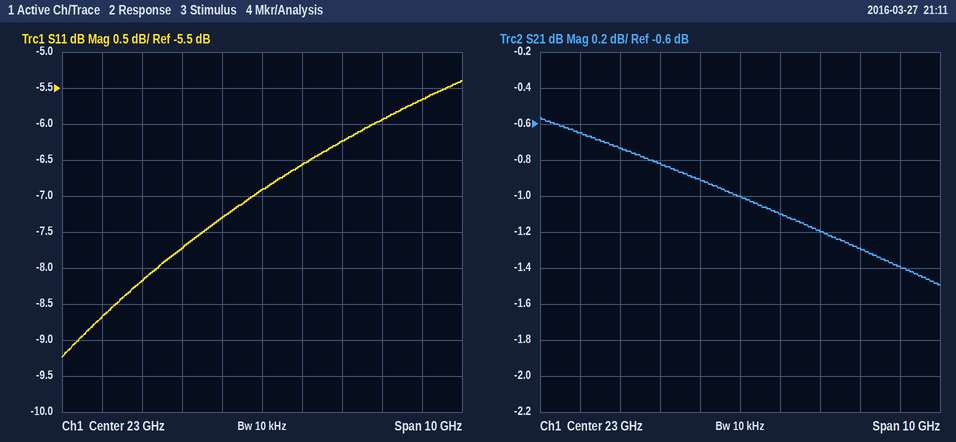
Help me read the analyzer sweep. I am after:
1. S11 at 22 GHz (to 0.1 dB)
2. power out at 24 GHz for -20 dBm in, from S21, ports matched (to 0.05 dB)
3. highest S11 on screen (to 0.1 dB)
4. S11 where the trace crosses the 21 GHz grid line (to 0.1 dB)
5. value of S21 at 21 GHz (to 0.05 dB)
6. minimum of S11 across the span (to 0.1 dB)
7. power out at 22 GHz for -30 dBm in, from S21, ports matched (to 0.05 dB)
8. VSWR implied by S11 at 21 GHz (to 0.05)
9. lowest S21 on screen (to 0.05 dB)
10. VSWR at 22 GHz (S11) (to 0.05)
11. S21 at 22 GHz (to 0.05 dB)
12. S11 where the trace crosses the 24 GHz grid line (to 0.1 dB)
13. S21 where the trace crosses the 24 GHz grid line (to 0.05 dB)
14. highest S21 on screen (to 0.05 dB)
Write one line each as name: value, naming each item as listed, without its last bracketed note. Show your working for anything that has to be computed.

S11 at 22 GHz: -7.3 dB
power out at 24 GHz for -20 dBm in, from S21, ports matched: -20 dBm + (-1.10 dB) = -21.10 dBm
highest S11 on screen: -5.4 dB
S11 where the trace crosses the 21 GHz grid line: -7.7 dB
value of S21 at 21 GHz: -0.80 dB
minimum of S11 across the span: -9.2 dB
power out at 22 GHz for -30 dBm in, from S21, ports matched: -30 dBm + (-0.90 dB) = -30.90 dBm
VSWR implied by S11 at 21 GHz: |Γ| = 10^(-7.7/20) = 0.4121; VSWR = (1 + 0.4121)/(1 − 0.4121) ≈ 2.40
lowest S21 on screen: -1.50 dB
VSWR at 22 GHz (S11): |Γ| = 10^(-7.3/20) = 0.4315; VSWR = (1 + 0.4315)/(1 − 0.4315) ≈ 2.52, so 2.50 to the nearest 0.05
S21 at 22 GHz: -0.90 dB
S11 where the trace crosses the 24 GHz grid line: -6.6 dB
S21 where the trace crosses the 24 GHz grid line: -1.10 dB
highest S21 on screen: -0.55 dB
